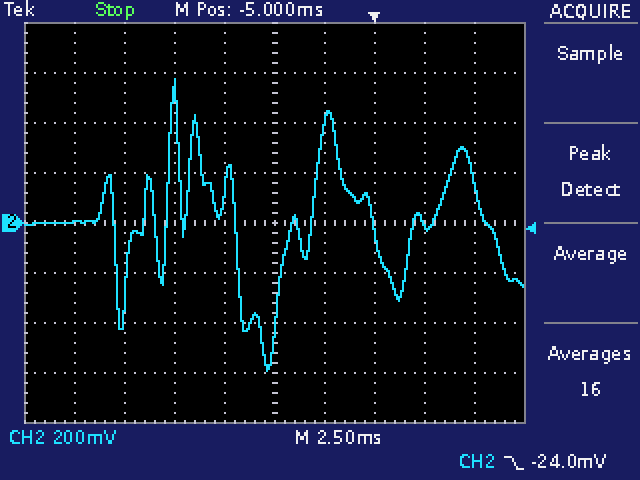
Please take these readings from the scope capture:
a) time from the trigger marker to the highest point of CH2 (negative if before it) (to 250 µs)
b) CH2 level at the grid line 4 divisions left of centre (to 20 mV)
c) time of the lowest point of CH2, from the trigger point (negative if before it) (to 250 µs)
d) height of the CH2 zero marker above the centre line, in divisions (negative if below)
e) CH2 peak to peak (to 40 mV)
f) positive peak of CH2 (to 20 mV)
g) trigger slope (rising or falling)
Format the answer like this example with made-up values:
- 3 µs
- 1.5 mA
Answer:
- -10.00 ms
- 0 mV
- -5.25 ms
- 0.0 div
- 1.16 V
- 580 mV
- falling
